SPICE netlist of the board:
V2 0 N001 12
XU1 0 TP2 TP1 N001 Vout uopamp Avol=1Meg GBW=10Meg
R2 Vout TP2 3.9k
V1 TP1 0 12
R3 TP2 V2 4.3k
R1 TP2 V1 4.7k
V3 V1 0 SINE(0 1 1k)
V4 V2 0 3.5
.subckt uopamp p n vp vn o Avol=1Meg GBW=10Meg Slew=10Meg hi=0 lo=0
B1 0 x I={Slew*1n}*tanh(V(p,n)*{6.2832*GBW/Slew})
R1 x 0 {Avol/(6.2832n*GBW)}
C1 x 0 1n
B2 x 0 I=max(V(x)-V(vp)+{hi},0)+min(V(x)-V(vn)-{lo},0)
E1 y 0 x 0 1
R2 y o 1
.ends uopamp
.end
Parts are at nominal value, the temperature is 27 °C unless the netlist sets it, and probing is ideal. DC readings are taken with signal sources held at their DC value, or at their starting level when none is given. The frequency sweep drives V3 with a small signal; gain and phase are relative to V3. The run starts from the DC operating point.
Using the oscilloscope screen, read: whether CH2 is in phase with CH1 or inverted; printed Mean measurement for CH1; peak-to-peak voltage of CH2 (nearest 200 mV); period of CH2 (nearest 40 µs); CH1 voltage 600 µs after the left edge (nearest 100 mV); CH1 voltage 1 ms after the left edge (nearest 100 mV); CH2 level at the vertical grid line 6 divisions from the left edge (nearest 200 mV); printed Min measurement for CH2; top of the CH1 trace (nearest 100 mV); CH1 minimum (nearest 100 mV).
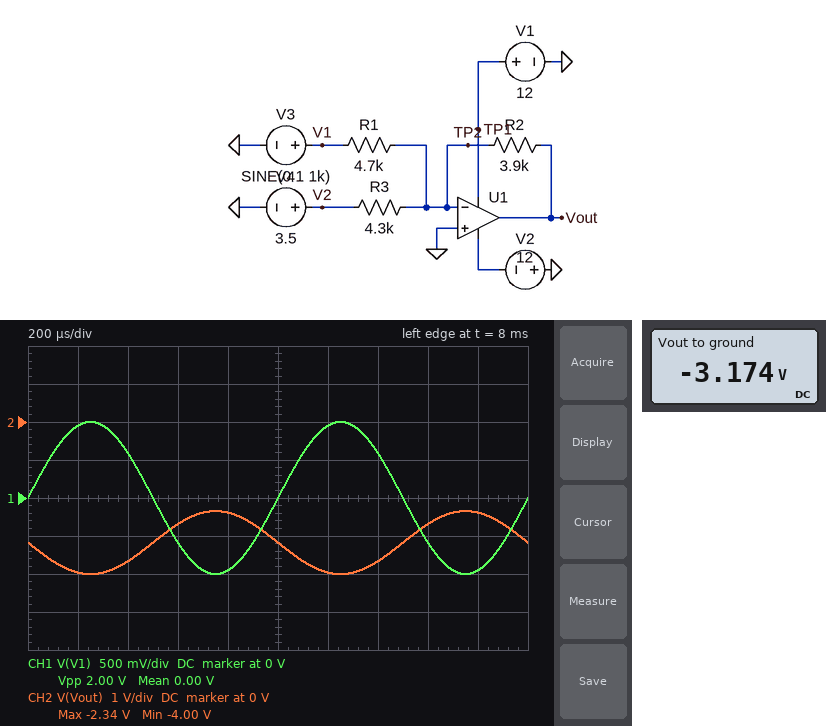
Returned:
inverted
0.00 V
1.6 V
1.00 ms
-600 mV
0 V
-4.0 V
-4.00 V
1.0 V
-1.0 V
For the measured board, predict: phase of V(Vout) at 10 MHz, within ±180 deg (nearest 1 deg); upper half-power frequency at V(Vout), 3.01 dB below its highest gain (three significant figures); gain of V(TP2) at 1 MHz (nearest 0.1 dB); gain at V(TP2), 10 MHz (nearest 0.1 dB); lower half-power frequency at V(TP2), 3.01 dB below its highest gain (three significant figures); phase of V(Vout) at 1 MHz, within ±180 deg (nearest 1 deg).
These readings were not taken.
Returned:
110 deg
3.65 MHz
-21.9 dB
-10.9 dB
3.65 MHz
165 deg
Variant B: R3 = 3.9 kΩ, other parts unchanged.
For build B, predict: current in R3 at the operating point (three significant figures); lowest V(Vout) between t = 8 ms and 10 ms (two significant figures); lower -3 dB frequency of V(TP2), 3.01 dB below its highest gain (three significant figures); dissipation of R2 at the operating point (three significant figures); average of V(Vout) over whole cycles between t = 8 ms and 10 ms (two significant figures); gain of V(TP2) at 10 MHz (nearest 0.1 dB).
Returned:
897 µA
-4.3 V
3.53 MHz
3.14 mW
-3.5 V
-11.2 dB
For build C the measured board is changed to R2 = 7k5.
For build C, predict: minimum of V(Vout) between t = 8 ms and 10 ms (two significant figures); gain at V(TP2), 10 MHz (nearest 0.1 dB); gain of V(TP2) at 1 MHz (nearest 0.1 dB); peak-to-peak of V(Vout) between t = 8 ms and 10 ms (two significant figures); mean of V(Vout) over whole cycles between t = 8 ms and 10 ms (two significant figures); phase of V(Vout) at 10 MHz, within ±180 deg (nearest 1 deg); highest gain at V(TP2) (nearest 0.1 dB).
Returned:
-7.7 V
-8.9 dB
-16.7 dB
3.2 V
-6.1 V
103 deg
-8.7 dB
